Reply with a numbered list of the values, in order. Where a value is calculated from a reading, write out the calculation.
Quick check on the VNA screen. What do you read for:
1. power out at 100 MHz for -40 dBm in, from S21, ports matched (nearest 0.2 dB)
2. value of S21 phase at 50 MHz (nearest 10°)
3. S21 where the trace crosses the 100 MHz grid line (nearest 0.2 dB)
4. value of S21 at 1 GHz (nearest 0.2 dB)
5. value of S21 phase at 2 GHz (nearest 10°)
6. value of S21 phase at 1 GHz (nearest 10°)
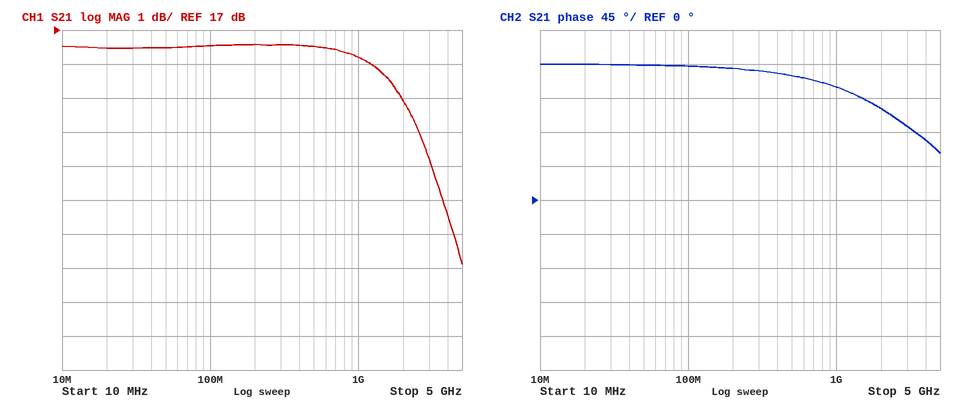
1. -40 dBm + (16.6 dB) = -23.4 dBm
2. 180°
3. 16.6 dB
4. 16.2 dB
5. 120°
6. 150°
